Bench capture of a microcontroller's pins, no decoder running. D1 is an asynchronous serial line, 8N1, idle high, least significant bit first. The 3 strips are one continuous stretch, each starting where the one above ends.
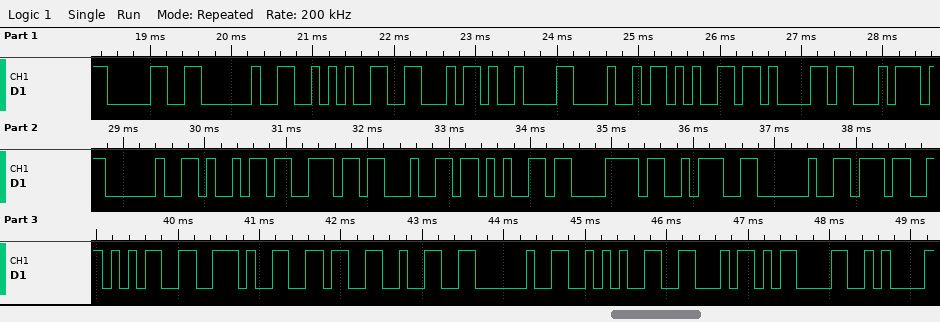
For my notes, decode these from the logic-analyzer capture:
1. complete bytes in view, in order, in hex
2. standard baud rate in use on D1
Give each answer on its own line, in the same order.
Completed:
30 20 2A 46 09 48 65 61 74 20 69 6E 64 65 78 3A 20 37 35 2E 36 32 20 2A 46 0D 0A
9600 baud
